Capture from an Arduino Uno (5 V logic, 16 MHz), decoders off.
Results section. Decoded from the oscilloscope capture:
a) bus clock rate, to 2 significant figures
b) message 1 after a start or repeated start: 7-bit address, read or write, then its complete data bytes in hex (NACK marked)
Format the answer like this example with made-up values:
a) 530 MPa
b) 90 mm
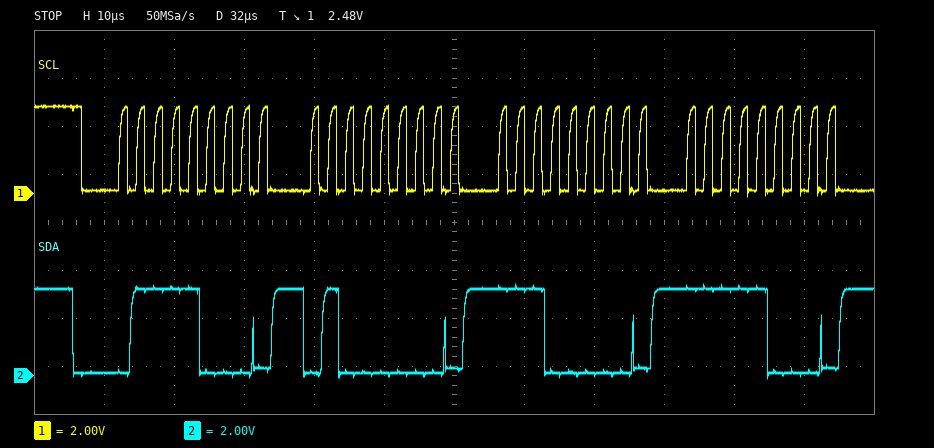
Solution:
a) 400 kHz
b) 0x3C write: 40 E0 F8
